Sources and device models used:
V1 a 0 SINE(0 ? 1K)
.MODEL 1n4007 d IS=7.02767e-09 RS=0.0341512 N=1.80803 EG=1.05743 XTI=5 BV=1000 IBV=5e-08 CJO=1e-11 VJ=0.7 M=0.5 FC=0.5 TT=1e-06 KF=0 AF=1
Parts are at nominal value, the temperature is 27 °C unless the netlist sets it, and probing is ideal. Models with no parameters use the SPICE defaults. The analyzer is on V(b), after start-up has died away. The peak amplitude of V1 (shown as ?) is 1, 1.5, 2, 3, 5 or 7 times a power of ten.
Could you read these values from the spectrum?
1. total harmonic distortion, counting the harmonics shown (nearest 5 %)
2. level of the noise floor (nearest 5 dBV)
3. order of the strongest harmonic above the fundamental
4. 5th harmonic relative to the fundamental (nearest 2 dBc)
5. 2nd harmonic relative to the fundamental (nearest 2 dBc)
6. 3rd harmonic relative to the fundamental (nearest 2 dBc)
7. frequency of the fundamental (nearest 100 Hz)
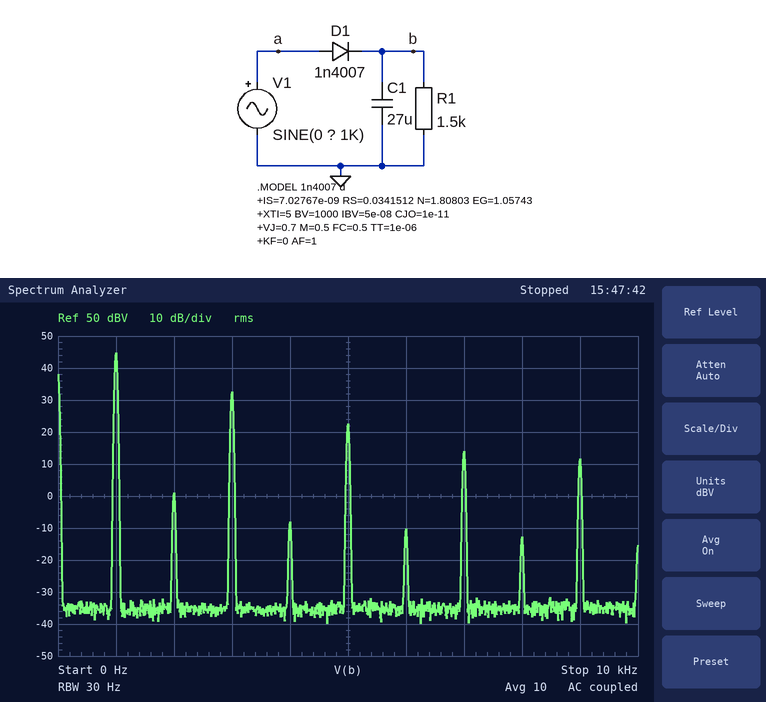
25 %
-35 dBV
3
-22 dBc
-44 dBc
-12 dBc
1.0 kHz
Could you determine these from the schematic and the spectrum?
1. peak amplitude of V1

700 V
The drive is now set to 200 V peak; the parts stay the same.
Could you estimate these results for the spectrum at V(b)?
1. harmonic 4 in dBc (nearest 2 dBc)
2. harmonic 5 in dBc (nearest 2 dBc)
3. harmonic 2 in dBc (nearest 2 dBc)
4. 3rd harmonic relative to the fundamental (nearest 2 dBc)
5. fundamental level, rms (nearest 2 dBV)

-12 dBc
-14 dBc
-6 dBc
-10 dBc
0 dBV
